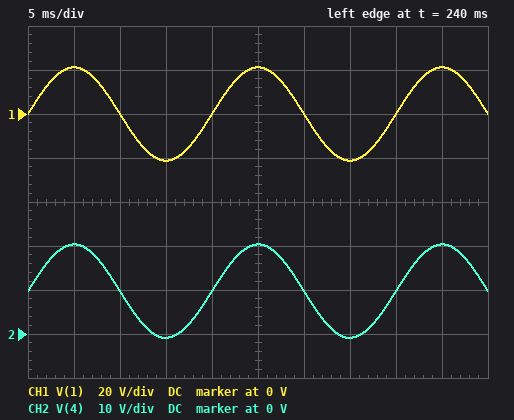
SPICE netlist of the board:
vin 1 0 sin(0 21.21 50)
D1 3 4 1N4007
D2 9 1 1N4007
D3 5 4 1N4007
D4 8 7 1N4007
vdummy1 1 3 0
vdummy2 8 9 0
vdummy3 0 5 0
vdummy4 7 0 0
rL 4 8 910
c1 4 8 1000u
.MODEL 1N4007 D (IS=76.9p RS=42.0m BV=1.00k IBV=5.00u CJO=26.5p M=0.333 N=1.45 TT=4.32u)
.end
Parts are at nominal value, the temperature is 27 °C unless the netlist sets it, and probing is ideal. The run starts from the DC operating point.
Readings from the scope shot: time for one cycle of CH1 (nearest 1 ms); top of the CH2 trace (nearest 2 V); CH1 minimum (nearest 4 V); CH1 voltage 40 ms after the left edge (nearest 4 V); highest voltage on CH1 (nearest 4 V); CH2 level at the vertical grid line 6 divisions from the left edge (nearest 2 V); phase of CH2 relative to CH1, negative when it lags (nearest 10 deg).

20 ms
20 V
-20 V
0 V
20 V
10 V
0 deg
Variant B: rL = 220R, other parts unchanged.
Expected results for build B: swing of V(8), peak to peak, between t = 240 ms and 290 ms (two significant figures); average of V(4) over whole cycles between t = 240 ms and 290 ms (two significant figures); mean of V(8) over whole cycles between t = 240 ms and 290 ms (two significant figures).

21 V
9.6 V
-9.6 V
